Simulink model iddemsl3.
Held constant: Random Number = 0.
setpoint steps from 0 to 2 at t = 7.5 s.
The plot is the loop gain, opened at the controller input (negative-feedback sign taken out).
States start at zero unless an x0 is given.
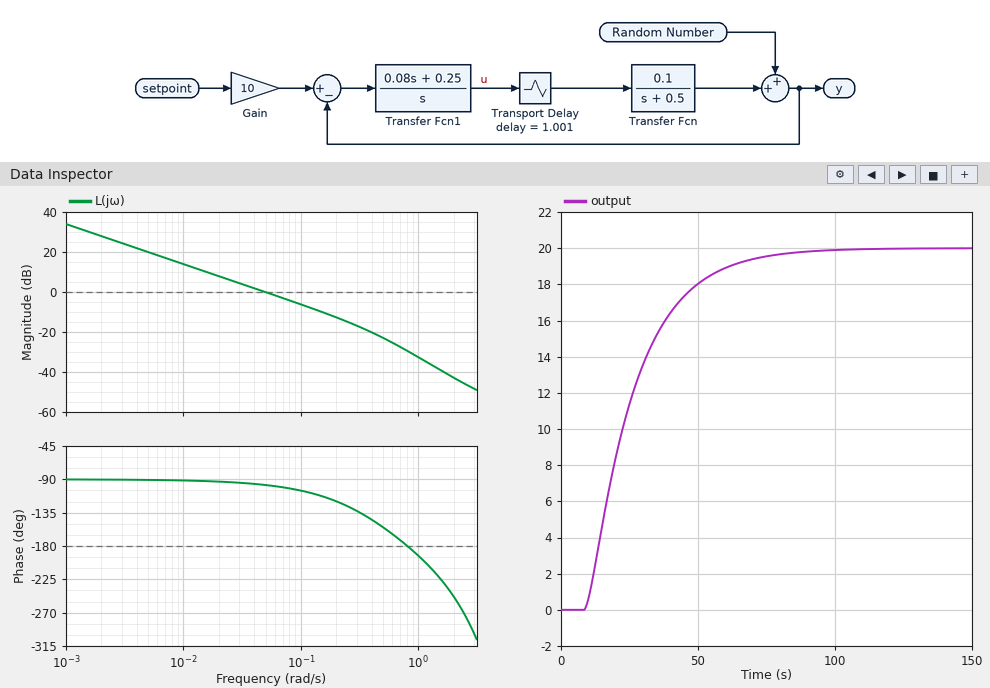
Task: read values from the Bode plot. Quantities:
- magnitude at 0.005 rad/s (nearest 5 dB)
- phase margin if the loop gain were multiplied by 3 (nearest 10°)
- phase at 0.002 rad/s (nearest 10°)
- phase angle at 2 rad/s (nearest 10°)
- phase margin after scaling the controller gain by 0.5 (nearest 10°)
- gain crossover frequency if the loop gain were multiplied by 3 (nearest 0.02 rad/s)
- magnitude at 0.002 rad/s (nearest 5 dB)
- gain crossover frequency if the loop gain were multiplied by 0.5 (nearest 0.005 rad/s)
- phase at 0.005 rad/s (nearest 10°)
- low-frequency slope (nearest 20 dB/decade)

20 dB
70°
-90°
-250°
90°
0.14 rad/s
30 dB
0.025 rad/s
-90°
-20 dB/decade
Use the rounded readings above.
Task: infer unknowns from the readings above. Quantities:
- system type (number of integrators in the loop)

1
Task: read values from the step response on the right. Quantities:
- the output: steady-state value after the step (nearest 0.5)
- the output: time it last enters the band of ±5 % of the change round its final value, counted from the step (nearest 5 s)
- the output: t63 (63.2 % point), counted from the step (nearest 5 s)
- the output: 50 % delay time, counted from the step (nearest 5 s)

20.0
55 s
20 s
15 s
